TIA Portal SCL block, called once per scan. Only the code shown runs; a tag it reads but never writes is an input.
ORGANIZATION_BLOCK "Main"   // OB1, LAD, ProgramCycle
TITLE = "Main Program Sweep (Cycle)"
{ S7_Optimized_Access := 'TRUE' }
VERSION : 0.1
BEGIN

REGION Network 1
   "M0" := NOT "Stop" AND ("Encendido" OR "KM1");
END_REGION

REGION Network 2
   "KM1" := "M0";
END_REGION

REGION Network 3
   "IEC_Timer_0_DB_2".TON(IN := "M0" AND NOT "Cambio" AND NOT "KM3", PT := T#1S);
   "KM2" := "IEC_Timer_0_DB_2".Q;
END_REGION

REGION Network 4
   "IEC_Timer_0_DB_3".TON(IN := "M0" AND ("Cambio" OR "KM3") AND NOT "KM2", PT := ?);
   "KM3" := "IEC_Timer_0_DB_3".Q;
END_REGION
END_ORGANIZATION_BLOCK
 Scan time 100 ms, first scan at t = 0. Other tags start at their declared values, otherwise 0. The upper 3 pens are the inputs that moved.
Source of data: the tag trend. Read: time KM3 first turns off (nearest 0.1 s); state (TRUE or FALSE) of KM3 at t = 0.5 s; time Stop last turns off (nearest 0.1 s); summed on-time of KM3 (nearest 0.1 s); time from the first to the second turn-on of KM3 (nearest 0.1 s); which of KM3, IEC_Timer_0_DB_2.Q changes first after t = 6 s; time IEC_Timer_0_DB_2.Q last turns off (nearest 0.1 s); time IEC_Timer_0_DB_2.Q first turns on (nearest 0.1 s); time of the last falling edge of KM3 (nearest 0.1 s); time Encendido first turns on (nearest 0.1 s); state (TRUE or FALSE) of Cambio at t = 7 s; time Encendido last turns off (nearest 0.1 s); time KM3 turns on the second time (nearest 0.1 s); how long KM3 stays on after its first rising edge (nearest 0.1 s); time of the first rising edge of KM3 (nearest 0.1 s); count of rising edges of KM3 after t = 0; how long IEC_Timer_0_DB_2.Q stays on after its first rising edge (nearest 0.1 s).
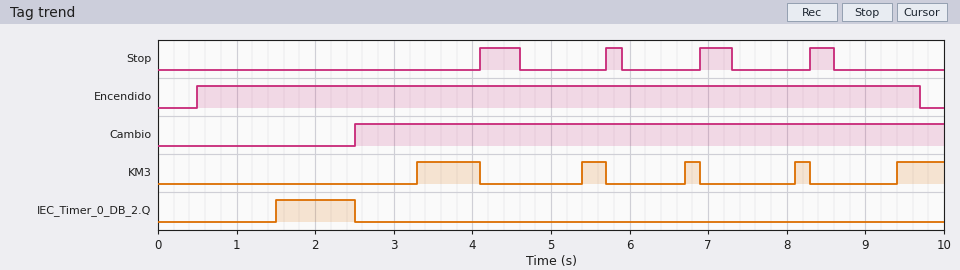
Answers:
4.1 s
FALSE
8.6 s
2.1 s
2.1 s
KM3
2.5 s
1.5 s
8.3 s
0.5 s
TRUE
9.7 s
5.4 s
0.8 s
3.3 s
5
1.0 s
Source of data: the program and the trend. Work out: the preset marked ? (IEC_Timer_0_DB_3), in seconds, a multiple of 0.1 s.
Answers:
0.8 s
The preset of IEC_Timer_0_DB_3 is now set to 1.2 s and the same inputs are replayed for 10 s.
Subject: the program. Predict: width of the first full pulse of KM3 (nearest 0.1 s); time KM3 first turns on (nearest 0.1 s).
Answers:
0.4 s
3.7 s
